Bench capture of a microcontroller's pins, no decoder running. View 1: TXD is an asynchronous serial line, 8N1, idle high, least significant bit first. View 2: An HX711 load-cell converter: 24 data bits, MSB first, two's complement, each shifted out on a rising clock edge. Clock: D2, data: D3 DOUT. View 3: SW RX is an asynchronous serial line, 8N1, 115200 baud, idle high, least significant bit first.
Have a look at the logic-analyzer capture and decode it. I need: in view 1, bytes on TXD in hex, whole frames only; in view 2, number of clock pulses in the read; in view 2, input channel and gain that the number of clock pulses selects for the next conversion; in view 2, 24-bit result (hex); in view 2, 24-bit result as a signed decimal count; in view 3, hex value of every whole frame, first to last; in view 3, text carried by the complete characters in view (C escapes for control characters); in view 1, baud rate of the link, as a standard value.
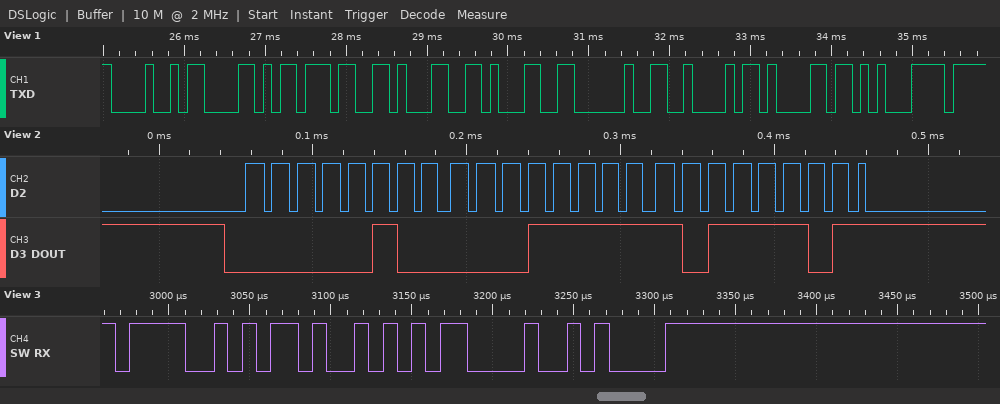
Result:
48 58 37 31 31 20 42 61 C5
25
channel A, gain 128
0x041FBD
270269
4F 4B 0D 0A
"OK\r\n"
9600 baud
